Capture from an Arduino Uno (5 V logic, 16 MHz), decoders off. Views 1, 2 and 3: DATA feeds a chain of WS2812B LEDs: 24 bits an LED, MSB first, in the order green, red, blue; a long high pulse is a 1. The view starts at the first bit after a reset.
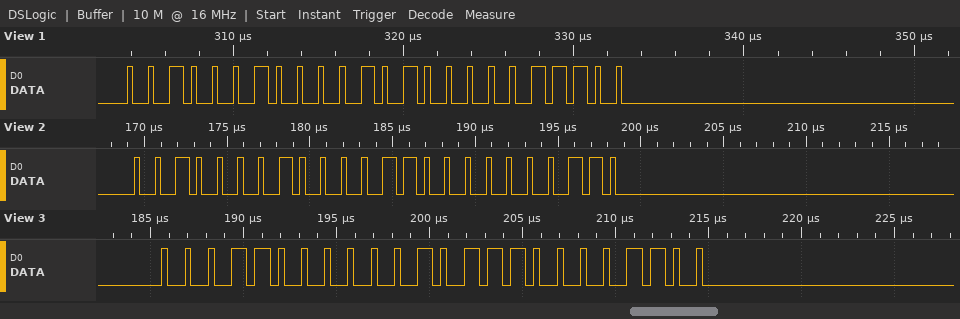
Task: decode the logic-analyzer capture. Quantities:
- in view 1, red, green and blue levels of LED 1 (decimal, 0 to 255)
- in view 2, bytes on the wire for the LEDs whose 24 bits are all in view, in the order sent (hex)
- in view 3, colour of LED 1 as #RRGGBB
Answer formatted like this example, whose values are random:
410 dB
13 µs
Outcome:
20, 34, 28
21 0C 06
#17180C
